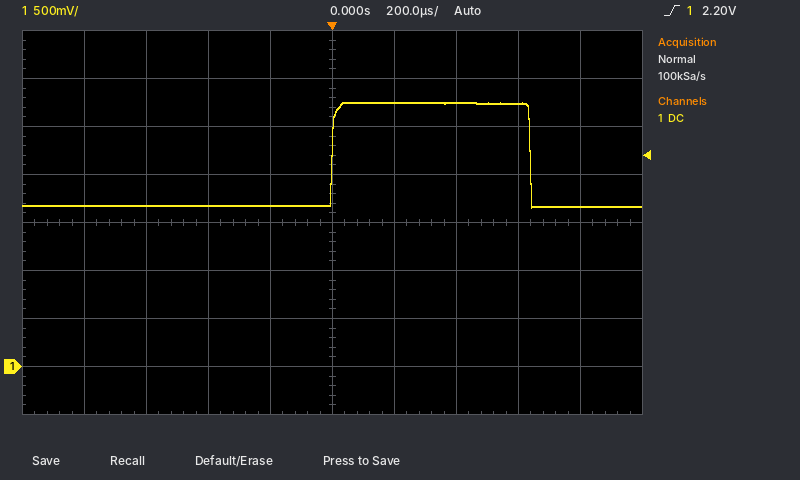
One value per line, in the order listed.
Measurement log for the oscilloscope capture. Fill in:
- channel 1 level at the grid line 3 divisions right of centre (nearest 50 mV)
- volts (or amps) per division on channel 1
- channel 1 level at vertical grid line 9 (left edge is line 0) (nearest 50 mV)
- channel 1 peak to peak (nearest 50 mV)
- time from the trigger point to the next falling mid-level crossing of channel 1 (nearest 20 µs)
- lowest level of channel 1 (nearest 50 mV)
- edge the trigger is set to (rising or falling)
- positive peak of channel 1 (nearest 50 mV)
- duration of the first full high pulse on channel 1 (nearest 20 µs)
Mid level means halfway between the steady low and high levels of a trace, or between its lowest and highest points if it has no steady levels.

2.75 V
500 mV
1.65 V
1.10 V
640 µs
1.65 V
rising
2.75 V
640 µs
